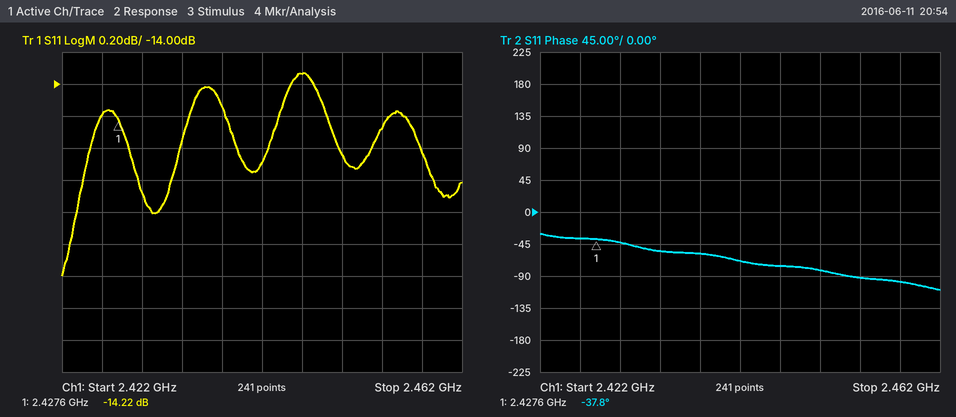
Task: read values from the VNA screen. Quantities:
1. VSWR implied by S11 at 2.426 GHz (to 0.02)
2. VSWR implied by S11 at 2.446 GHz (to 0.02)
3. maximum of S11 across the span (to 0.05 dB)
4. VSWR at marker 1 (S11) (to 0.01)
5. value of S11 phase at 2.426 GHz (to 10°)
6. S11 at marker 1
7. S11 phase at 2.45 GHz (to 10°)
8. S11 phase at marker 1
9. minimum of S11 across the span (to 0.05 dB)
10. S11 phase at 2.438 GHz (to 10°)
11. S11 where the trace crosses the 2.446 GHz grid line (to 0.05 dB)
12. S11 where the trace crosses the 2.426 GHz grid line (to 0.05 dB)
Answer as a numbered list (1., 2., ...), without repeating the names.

1. 1.48
2. 1.50
3. -13.95 dB
4. 1.48
5. -40°
6. -14.22 dB
7. -80°
8. -37.8°
9. -15.20 dB
10. -60°
11. -13.95 dB
12. -14.20 dB
